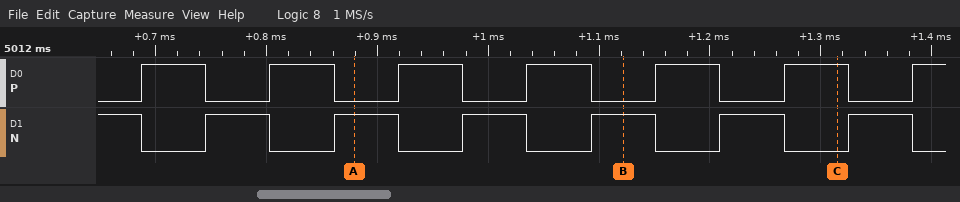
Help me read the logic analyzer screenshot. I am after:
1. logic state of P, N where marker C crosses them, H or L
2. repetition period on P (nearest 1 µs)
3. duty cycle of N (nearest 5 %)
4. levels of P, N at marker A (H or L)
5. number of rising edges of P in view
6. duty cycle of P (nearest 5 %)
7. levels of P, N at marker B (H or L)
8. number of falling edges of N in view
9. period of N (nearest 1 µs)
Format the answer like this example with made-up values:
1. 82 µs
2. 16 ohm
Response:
1. P=H, N=L
2. 116 µs
3. 50 %
4. P=L, N=H
5. 7
6. 50 %
7. P=L, N=H
8. 7
9. 116 µs
